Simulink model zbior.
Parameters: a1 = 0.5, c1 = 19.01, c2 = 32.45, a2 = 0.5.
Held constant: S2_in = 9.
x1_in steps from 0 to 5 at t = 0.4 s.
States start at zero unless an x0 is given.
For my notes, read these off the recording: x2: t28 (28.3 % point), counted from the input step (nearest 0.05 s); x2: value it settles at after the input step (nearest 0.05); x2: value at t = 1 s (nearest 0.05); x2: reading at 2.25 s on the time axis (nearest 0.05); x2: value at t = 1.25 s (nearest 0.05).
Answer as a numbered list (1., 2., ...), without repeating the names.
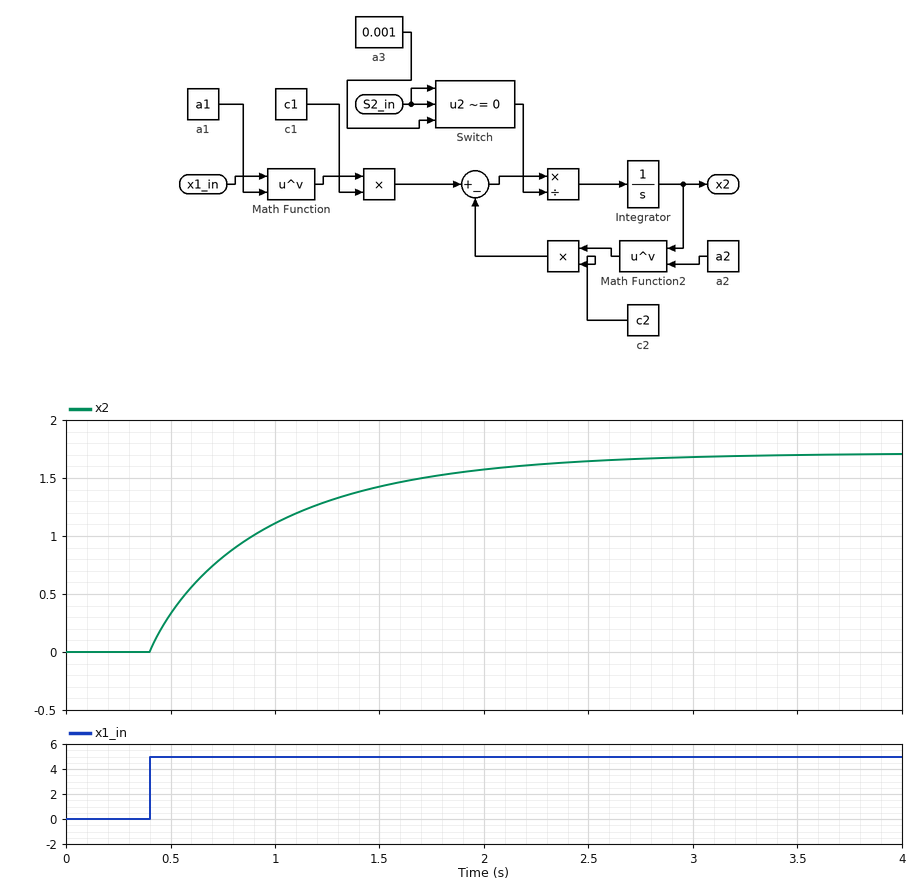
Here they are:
1. 0.15 s
2. 1.70
3. 1.10
4. 1.60
5. 1.30
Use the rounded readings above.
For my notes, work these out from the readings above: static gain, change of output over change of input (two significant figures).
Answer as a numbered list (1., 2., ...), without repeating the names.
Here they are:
1. 0.34
